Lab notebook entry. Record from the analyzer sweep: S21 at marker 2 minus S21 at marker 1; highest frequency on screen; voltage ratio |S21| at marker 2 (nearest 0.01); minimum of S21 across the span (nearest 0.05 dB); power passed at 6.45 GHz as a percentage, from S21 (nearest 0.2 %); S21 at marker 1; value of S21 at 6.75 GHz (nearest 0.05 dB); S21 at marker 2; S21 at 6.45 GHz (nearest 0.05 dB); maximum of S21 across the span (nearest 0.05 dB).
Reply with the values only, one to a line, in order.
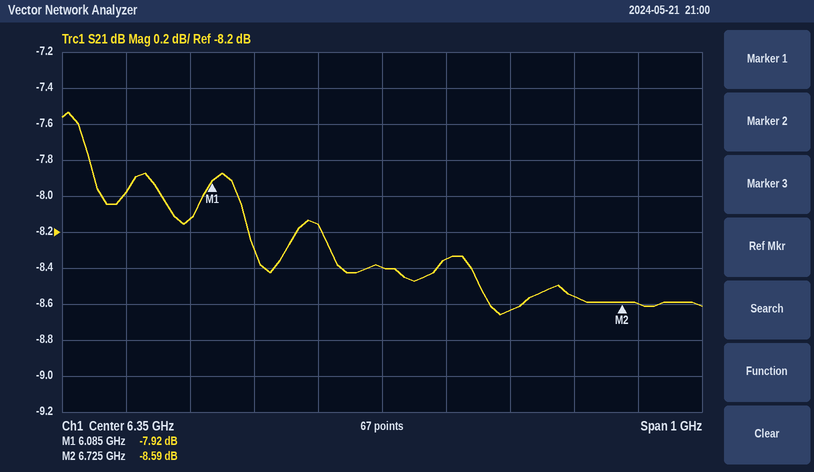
-0.67 dB
6.85 GHz
0.37
-8.65 dB
14.6 %
-7.92 dB
-8.60 dB
-8.59 dB
-8.35 dB
-7.55 dB
